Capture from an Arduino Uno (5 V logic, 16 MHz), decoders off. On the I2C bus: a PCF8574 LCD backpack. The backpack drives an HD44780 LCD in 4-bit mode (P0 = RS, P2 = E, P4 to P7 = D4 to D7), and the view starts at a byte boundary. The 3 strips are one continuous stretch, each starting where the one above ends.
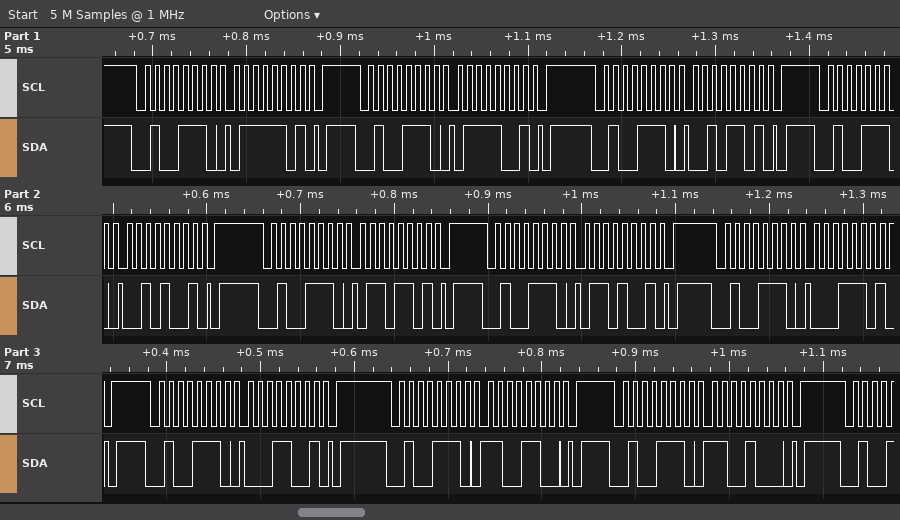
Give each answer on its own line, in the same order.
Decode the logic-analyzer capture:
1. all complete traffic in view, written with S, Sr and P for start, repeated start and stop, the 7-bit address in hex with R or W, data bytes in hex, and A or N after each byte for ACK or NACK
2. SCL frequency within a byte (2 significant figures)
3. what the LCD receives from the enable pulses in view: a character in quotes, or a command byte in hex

S 27W A 7D A P S 27W A 79 A P S 27W A 2D A P S 27W A 29 A P S 27W A 6D A P S 27W A 69 A P S 27W A 1D A P S 27W A 19 A P S 27W A CC A P S 27W A C8 A P
100 kHz
'r' 'a'
